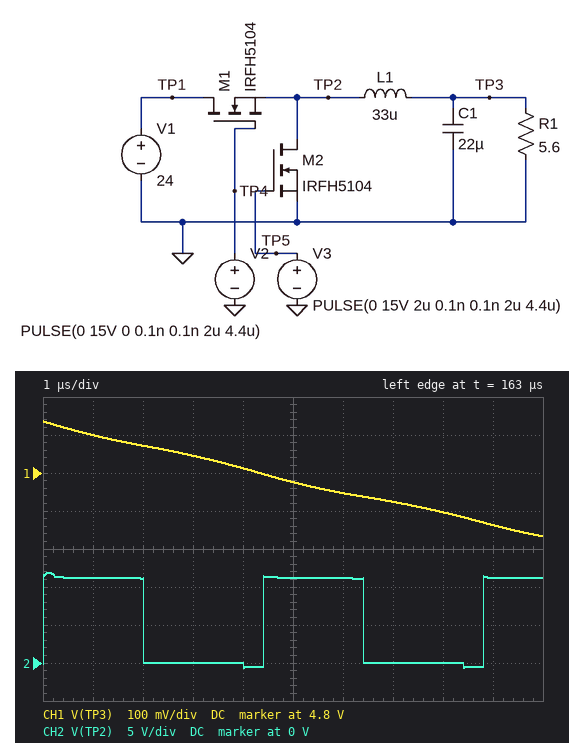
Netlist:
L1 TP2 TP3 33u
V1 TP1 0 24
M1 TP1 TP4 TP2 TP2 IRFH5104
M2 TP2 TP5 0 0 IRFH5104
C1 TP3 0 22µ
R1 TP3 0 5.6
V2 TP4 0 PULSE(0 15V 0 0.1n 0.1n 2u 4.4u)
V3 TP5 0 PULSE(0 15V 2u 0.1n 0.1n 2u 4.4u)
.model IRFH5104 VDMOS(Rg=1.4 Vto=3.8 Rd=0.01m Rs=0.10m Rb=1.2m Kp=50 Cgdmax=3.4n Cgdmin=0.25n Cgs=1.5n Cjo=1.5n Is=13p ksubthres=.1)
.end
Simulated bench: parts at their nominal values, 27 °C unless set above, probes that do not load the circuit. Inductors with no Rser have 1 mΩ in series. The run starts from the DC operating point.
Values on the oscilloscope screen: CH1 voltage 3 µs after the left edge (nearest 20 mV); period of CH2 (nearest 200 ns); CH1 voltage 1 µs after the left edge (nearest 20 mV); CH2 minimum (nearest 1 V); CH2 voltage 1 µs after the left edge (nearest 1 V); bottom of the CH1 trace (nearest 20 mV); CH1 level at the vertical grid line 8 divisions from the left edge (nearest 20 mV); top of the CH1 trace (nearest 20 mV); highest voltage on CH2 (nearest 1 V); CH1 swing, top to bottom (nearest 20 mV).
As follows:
4.84 V
4.4 µs
4.90 V
-1 V
11 V
4.64 V
4.70 V
4.94 V
12 V
300 mV
